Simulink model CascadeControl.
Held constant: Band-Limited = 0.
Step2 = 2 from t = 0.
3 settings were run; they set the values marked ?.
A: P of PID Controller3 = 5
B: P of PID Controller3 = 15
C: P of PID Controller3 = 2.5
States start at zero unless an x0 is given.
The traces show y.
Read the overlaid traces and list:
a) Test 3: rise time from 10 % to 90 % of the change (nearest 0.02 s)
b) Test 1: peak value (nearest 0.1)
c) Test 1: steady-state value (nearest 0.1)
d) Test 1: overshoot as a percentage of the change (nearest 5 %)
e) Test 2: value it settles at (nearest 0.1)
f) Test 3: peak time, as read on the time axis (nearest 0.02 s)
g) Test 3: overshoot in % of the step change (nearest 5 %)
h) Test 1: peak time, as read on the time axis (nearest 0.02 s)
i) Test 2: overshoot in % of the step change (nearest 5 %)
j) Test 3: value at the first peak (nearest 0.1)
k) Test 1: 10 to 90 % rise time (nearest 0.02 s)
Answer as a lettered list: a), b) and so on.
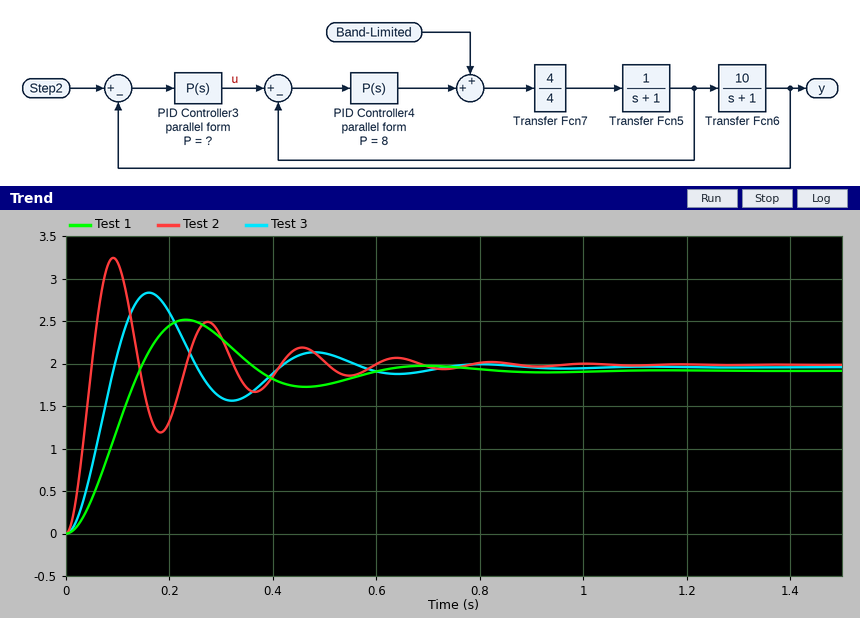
a) 0.06 s
b) 2.5
c) 1.9
d) 30 %
e) 2.0
f) 0.16 s
g) 45 %
h) 0.24 s
i) 65 %
j) 2.8
k) 0.10 s
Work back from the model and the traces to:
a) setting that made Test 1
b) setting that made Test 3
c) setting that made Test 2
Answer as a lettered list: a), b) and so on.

a) C
b) A
c) B
